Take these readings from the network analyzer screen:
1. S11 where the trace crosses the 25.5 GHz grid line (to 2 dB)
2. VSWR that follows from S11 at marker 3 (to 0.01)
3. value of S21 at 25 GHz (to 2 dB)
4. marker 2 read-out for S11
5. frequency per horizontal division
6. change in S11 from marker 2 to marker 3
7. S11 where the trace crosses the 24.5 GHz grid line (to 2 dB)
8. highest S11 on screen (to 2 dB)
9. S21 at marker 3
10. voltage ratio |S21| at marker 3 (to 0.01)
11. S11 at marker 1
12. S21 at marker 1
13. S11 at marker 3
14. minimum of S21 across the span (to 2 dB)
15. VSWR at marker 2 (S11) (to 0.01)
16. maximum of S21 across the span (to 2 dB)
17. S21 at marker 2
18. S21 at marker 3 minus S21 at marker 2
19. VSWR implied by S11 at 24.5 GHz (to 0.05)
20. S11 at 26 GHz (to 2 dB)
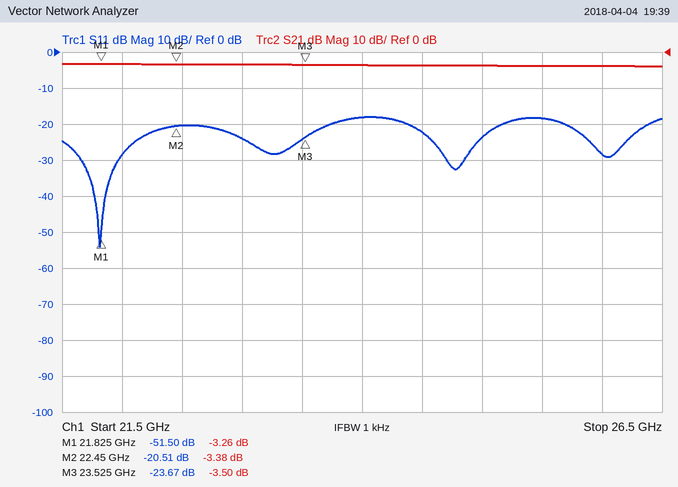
-18 dB
1.14
-4 dB
-20.51 dB
500 MHz
-3.16 dB
-22 dB
-18 dB
-3.50 dB
0.67
-51.50 dB
-3.26 dB
-23.67 dB
-4 dB
1.21
-4 dB
-3.38 dB
-0.12 dB
1.15
-28 dB
